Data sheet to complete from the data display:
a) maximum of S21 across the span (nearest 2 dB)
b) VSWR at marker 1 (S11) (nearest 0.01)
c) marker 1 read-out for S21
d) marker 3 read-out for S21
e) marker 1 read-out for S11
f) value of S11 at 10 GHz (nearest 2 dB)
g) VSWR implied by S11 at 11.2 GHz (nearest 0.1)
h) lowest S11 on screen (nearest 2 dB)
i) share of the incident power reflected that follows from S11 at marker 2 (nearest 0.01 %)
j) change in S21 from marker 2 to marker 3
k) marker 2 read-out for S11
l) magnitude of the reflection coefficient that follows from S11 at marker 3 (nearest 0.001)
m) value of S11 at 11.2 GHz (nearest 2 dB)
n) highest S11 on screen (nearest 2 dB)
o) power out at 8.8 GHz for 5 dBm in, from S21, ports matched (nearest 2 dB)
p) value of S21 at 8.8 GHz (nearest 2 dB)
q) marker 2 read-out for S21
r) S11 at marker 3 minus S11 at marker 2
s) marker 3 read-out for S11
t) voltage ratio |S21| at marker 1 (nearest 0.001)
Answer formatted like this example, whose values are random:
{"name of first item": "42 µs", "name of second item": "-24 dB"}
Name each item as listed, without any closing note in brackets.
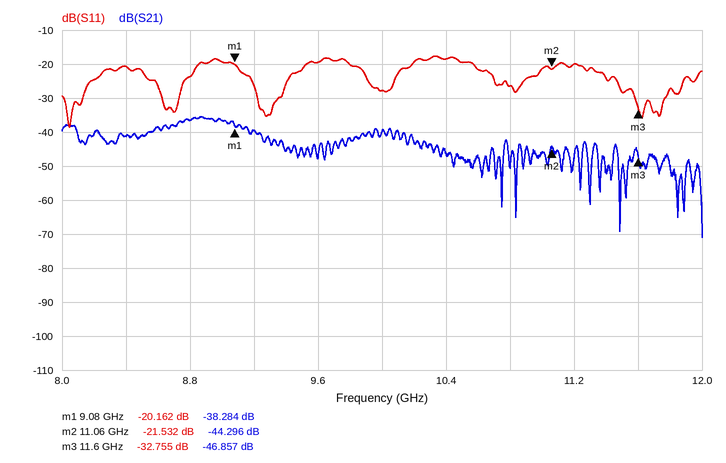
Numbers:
{"maximum of S21 across the span": "-36 dB", "VSWR at marker 1 (S11)": "1.22", "marker 1 read-out for S21": "-38.284 dB", "marker 3 read-out for S21": "-46.857 dB", "marker 1 read-out for S11": "-20.162 dB", "value of S11 at 10 GHz": "-28 dB", "VSWR implied by S11 at 11.2 GHz": "1.2", "lowest S11 on screen": "-38 dB", "share of the incident power reflected that follows from S11 at marker 2": "0.70 %", "change in S21 from marker 2 to marker 3": "-2.561 dB", "marker 2 read-out for S11": "-21.532 dB", "magnitude of the reflection coefficient that follows from S11 at marker 3": "0.023", "value of S11 at 11.2 GHz": "-20 dB", "highest S11 on screen": "-18 dB", "power out at 8.8 GHz for 5 dBm in, from S21, ports matched": "-32 dBm", "value of S21 at 8.8 GHz": "-36 dB", "marker 2 read-out for S21": "-44.296 dB", "S11 at marker 3 minus S11 at marker 2": "-11.223 dB", "marker 3 read-out for S11": "-32.755 dB", "voltage ratio |S21| at marker 1": "0.012"}
